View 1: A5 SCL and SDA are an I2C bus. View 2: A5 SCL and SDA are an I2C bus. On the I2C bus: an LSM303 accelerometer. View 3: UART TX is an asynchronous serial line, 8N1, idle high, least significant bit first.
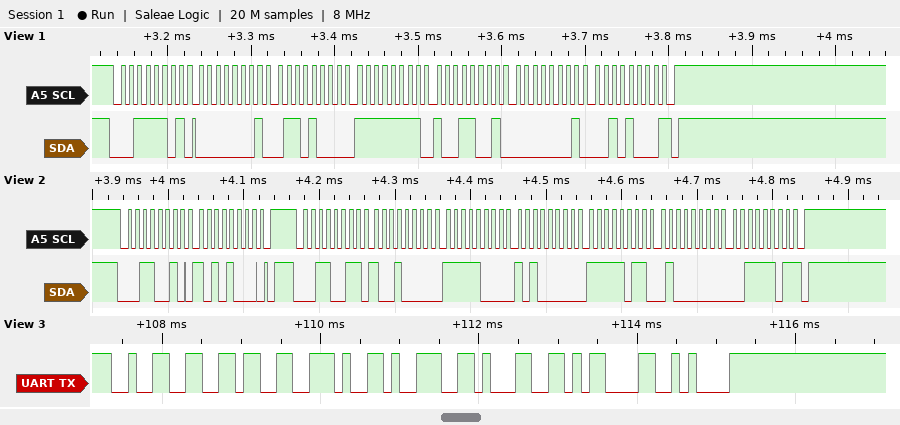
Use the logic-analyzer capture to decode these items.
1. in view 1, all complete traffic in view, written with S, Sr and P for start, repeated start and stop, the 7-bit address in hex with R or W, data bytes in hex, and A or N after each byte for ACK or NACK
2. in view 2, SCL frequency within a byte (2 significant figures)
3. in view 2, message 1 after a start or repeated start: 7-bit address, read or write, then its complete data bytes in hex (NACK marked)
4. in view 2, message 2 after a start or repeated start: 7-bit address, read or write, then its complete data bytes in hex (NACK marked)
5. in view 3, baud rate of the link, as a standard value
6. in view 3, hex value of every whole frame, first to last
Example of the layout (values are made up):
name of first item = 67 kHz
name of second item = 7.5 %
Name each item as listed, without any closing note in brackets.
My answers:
in view 1, all complete traffic in view, written with S, Sr and P for start, repeated start and stop, the 7-bit address in hex with R or W, data bytes in hex, and A or N after each byte for ACK or NACK = S 1ER A 01 A 68 A FF A 99 A 01 A 28 N P
in view 2, SCL frequency within a byte = 100 kHz
in view 2, message 1 after a start or repeated start: 7-bit address, read or write, then its complete data bytes in hex = 0x19 write: A8
in view 2, message 2 after a start or repeated start: 7-bit address, read or write, then its complete data bytes in hex = 0x19 read: 90 F8 A0 FB 40 3D NACK
in view 3, baud rate of the link, as a standard value = 9600 baud
in view 3, hex value of every whole frame, first to last = 32 36 2E 39 31 0D 0A
